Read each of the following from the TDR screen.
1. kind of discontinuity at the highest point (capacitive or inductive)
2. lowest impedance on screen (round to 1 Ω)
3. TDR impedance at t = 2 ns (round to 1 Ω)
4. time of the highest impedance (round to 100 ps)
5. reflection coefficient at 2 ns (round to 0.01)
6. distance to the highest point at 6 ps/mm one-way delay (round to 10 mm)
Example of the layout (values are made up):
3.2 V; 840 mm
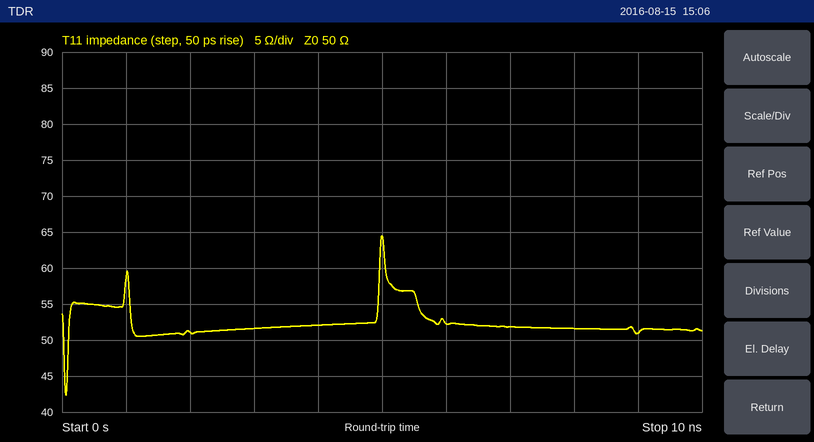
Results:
inductive; 42 Ω; 51 Ω; 5.0 ns; +0.01; 420 mm
